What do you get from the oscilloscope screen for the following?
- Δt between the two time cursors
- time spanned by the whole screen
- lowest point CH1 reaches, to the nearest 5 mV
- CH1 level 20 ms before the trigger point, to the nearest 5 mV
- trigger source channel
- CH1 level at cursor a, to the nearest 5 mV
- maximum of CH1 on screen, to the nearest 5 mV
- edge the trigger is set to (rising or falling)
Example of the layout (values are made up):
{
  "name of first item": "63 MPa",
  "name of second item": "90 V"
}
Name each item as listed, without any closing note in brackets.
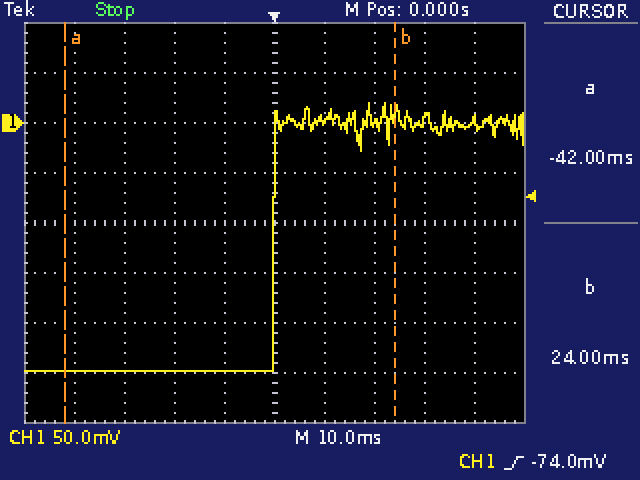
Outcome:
{
  "Δt between the two time cursors": "66 ms",
  "time spanned by the whole screen": "100 ms",
  "lowest point CH1 reaches, to the nearest 5 mV": "-250 mV",
  "CH1 level 20 ms before the trigger point, to the nearest 5 mV": "-250 mV",
  "trigger source channel": "CH1",
  "CH1 level at cursor a, to the nearest 5 mV": "-250 mV",
  "maximum of CH1 on screen, to the nearest 5 mV": "20 mV",
  "edge the trigger is set to": "rising"
}
